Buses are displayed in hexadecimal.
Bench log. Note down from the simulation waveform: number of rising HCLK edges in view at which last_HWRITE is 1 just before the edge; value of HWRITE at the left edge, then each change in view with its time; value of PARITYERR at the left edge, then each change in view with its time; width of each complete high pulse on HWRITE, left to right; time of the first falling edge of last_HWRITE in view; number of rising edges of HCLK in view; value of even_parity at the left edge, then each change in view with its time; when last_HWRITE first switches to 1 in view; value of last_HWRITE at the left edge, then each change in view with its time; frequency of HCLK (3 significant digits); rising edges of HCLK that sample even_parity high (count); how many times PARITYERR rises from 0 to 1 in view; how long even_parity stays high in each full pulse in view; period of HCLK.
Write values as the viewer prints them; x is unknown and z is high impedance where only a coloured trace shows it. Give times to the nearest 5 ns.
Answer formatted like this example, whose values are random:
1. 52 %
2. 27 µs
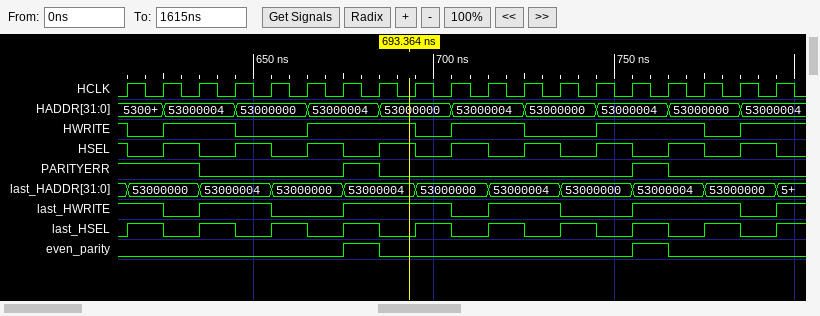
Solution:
1. 12
2. 1, 0 at 615 ns, 1 at 625 ns, 0 at 645 ns, 1 at 665 ns, 0 at 695 ns, 1 at 705 ns, 0 at 725 ns, 1 at 745 ns, 0 at 775 ns, 1 at 785 ns
3. 1, 0 at 635 ns, 1 at 675 ns, 0 at 685 ns, 1 at 755 ns, 0 at 765 ns
4. 20 ns, 30 ns, 20 ns, 30 ns
5. 625 ns
6. 19
7. 0, 1 at 675 ns, 0 at 685 ns, 1 at 755 ns, 0 at 765 ns
8. 635 ns
9. 1, 0 at 625 ns, 1 at 635 ns, 0 at 655 ns, 1 at 675 ns, 0 at 705 ns, 1 at 715 ns, 0 at 735 ns, 1 at 755 ns, 0 at 785 ns, 1 at 795 ns
10. 100 MHz
11. 2
12. 2
13. 10 ns, 10 ns
14. 10 ns
